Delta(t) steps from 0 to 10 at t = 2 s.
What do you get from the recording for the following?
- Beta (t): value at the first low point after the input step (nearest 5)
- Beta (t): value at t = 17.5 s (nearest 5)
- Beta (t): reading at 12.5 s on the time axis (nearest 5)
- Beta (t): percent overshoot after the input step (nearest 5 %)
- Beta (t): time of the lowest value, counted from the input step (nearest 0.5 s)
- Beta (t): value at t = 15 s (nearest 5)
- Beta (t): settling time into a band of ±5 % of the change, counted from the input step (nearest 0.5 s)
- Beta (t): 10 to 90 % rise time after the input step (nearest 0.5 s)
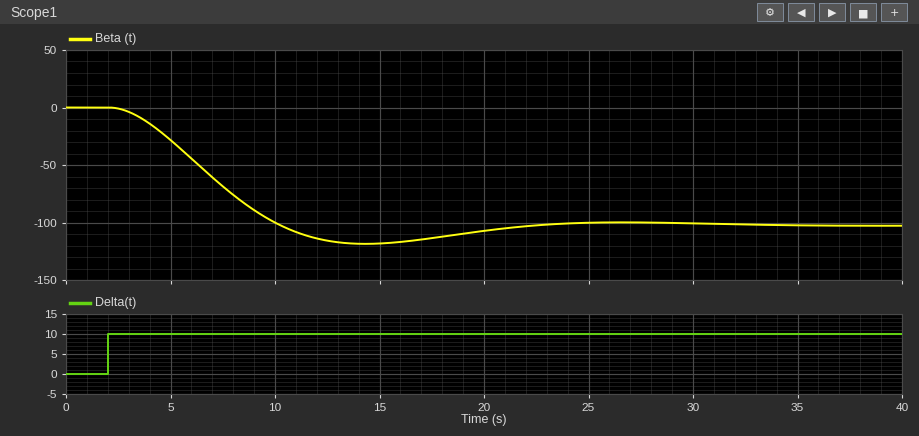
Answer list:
-120
-115
-115
15 %
12.5 s
-120
18.0 s
5.5 s
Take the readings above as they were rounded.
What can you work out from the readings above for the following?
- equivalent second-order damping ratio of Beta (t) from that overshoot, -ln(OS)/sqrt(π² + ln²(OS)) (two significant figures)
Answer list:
0.52
